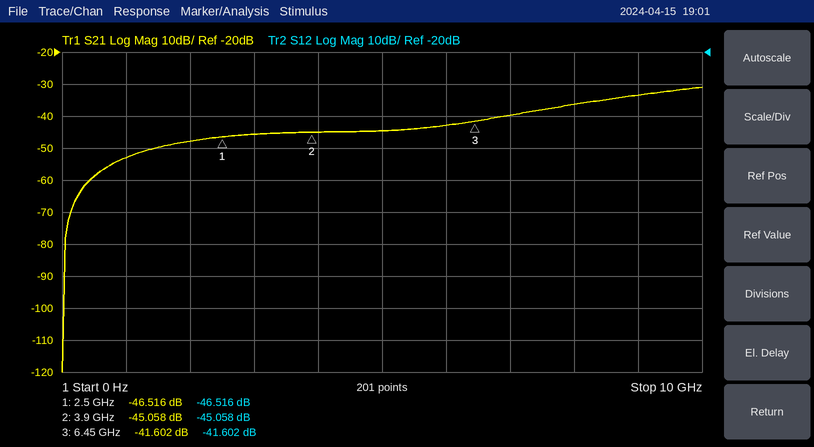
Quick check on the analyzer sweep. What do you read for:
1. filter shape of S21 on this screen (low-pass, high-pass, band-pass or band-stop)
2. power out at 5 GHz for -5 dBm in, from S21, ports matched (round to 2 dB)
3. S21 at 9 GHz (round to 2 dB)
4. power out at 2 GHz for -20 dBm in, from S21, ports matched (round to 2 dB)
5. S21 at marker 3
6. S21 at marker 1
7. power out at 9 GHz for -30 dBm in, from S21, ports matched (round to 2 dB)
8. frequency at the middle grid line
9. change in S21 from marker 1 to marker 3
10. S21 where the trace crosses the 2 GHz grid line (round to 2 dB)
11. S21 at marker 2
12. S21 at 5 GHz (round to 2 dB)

high-pass
-50 dBm
-34 dB
-68 dBm
-41.602 dB
-46.516 dB
-64 dBm
5 GHz
4.914 dB
-48 dB
-45.058 dB
-44 dB
